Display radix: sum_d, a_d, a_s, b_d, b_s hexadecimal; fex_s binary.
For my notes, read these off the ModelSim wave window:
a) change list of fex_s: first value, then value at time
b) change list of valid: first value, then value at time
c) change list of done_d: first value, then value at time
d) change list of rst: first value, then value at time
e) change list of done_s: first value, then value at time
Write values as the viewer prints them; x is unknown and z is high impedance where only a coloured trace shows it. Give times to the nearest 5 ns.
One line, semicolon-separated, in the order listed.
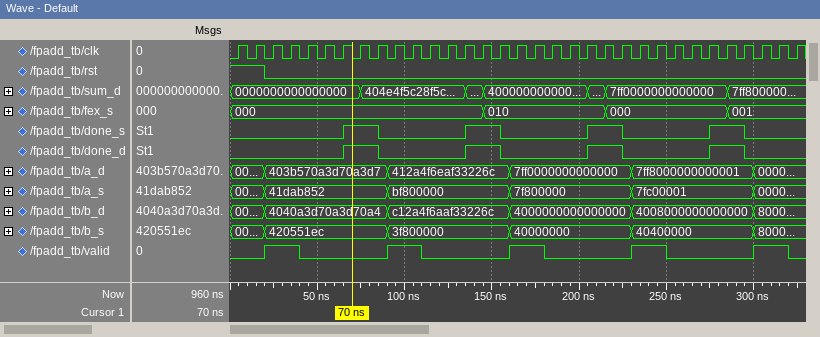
000, 010 at 145 ns, 000 at 215 ns, 001 at 285 ns; 0, 1 at 20 ns, 0 at 40 ns, 1 at 90 ns, 0 at 110 ns, 1 at 160 ns, 0 at 180 ns, 1 at 230 ns, 0 at 250 ns, 1 at 300 ns, 0 at 320 ns; 0, 1 at 65 ns, 0 at 85 ns, 1 at 135 ns, 0 at 155 ns, 1 at 205 ns, 0 at 225 ns, 1 at 275 ns, 0 at 295 ns; 1, 0 at 20 ns; 0, 1 at 65 ns, 0 at 85 ns, 1 at 135 ns, 0 at 155 ns, 1 at 205 ns, 0 at 225 ns, 1 at 275 ns, 0 at 295 ns
